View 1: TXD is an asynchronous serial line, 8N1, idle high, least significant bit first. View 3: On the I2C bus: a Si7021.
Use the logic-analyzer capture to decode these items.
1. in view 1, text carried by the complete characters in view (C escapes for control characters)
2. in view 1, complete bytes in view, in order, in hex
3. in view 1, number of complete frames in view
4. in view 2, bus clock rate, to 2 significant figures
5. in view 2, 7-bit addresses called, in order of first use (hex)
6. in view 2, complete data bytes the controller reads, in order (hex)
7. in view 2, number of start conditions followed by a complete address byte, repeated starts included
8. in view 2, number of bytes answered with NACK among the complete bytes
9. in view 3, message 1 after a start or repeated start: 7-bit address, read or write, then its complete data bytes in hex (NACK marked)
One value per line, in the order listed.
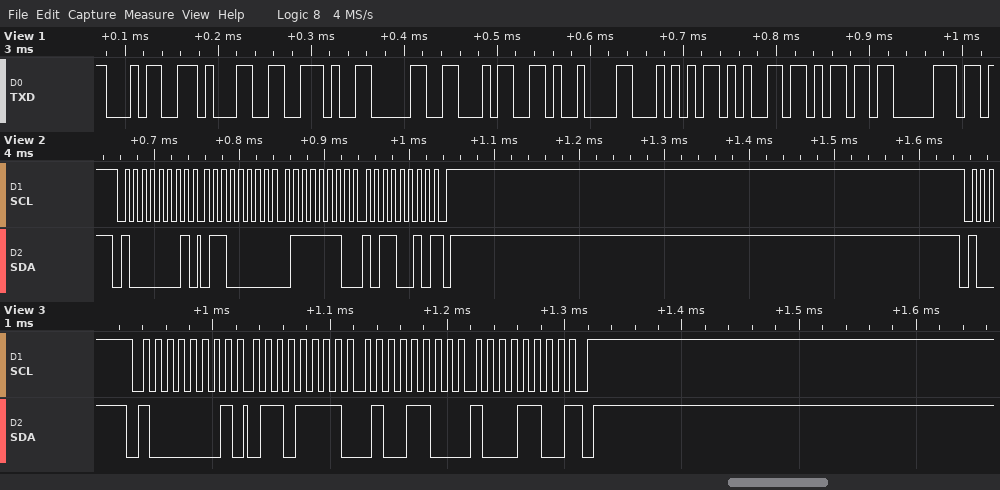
"41.04\tTemp"
34 31 2E 30 34 09 54 65 6D 70
10
100 kHz
0x40
60 7E B2
1
1
0x40 read: 6F 4C 8C NACK
